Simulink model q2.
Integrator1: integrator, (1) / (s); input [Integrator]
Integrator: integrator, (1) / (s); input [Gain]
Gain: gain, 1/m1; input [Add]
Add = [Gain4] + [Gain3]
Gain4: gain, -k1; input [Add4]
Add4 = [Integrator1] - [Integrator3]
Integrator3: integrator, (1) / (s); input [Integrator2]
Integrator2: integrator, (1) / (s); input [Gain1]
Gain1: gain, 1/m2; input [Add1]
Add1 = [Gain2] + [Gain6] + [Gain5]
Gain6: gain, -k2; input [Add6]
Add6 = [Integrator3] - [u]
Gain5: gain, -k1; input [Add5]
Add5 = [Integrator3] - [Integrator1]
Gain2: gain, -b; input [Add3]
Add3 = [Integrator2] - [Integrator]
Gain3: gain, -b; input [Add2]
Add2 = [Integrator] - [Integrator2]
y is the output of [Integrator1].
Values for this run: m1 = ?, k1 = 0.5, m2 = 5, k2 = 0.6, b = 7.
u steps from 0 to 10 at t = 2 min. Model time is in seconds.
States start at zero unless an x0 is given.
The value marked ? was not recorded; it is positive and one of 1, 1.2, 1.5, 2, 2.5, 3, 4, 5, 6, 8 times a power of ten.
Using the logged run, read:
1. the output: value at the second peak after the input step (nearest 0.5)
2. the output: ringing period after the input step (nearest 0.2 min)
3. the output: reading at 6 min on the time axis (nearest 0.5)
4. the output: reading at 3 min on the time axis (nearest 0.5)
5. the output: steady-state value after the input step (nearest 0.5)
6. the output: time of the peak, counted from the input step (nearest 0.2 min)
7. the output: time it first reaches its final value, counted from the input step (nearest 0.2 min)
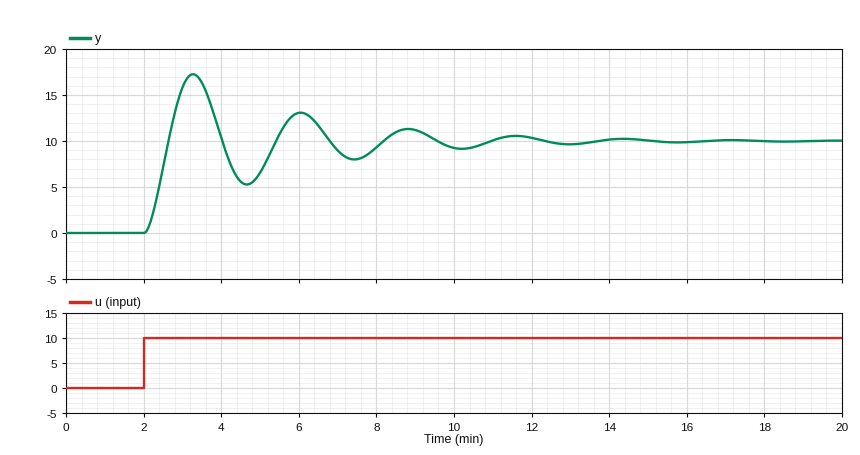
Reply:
13.0
2.8 min
13.0
16.0
10.0
1.2 min
0.6 min
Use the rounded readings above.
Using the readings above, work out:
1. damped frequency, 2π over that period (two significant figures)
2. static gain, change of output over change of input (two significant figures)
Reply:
2.2 rad/min
1.0
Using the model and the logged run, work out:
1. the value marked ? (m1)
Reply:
200
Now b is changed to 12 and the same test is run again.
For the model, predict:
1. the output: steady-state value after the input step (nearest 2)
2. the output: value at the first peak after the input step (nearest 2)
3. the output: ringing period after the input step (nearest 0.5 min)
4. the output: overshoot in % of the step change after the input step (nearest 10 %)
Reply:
10
16
2.5 min
70 %
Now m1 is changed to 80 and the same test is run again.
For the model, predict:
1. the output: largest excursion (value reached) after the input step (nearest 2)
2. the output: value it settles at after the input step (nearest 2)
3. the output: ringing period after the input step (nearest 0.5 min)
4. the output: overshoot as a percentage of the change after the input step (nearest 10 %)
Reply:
16
10
1.5 min
70 %
